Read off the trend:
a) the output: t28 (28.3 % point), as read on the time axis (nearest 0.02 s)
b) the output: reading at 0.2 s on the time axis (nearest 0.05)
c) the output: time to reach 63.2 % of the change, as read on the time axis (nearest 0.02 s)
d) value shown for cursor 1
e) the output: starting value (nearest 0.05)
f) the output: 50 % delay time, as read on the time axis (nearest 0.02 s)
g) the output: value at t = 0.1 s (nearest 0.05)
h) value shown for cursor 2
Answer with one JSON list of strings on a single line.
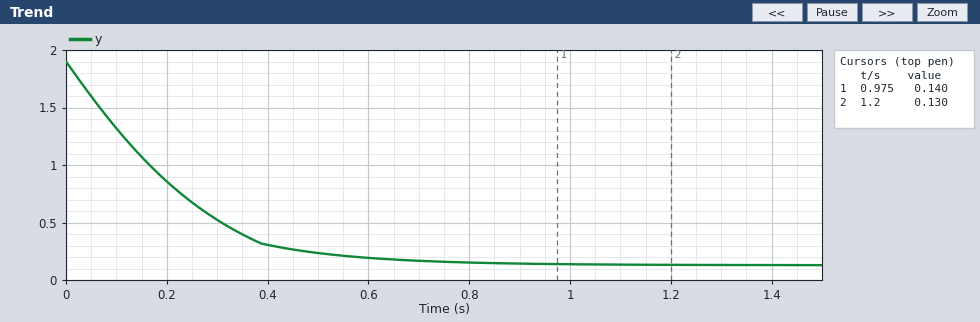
["0.08 s", "0.85", "0.22 s", "0.140", "1.90", "0.16 s", "1.30", "0.130"]
